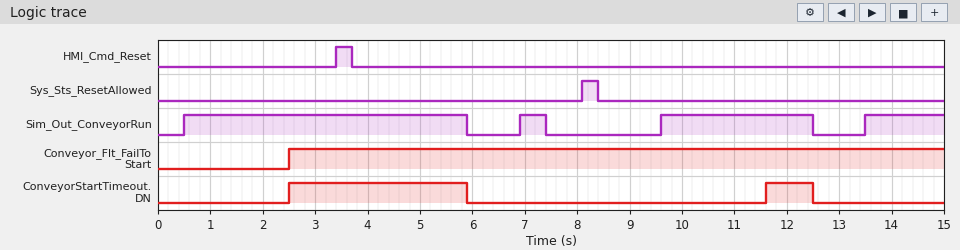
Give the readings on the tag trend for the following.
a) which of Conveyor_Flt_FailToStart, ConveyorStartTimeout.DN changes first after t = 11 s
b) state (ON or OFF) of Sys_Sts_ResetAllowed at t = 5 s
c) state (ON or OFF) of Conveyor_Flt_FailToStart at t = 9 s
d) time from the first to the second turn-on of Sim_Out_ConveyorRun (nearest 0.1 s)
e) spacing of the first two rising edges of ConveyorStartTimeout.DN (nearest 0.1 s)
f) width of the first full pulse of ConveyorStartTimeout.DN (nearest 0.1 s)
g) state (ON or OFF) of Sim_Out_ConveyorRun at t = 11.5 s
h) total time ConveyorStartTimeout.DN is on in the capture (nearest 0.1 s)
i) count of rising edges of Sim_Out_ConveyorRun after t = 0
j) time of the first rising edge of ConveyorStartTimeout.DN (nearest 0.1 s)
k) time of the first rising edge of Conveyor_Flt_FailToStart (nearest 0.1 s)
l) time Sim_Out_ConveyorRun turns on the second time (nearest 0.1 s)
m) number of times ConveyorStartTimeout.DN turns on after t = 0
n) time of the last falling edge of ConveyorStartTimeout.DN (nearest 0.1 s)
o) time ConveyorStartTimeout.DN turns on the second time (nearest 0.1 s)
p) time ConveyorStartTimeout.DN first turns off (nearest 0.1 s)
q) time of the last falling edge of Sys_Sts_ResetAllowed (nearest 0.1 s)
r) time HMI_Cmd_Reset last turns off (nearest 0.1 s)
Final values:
ConveyorStartTimeout.DN
OFF
ON
6.4 s
9.1 s
3.4 s
ON
4.3 s
4
2.5 s
2.5 s
6.9 s
2
12.5 s
11.6 s
5.9 s
8.4 s
3.7 s
